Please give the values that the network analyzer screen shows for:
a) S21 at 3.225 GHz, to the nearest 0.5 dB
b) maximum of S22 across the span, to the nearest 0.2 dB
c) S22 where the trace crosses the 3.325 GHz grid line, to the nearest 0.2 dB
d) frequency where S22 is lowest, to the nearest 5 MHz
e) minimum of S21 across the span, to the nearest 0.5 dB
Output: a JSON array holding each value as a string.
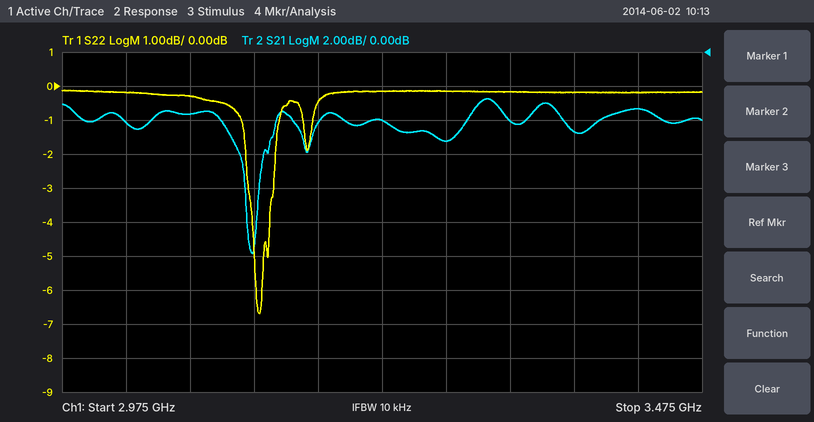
["-4.0 dB", "-0.2 dB", "-0.2 dB", "3.130 GHz", "-12.0 dB"]
